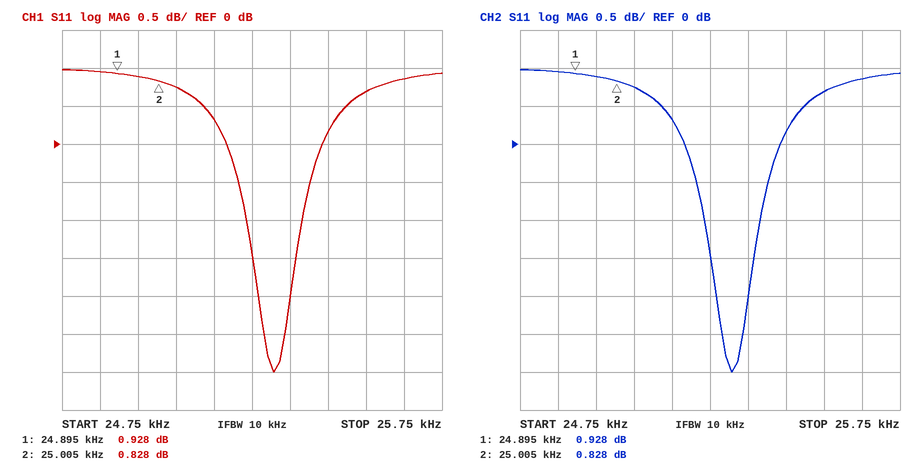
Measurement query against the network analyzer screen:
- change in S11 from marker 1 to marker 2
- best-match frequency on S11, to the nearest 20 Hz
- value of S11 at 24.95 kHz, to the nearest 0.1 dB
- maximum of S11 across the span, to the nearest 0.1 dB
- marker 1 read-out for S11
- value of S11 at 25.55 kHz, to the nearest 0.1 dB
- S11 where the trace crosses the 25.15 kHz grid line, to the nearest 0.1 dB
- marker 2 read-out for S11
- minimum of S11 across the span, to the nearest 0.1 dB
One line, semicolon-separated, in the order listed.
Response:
-0.100 dB; 25.30 kHz; 0.9 dB; 1.0 dB; 0.928 dB; 0.7 dB; 0.3 dB; 0.828 dB; -3.0 dB
